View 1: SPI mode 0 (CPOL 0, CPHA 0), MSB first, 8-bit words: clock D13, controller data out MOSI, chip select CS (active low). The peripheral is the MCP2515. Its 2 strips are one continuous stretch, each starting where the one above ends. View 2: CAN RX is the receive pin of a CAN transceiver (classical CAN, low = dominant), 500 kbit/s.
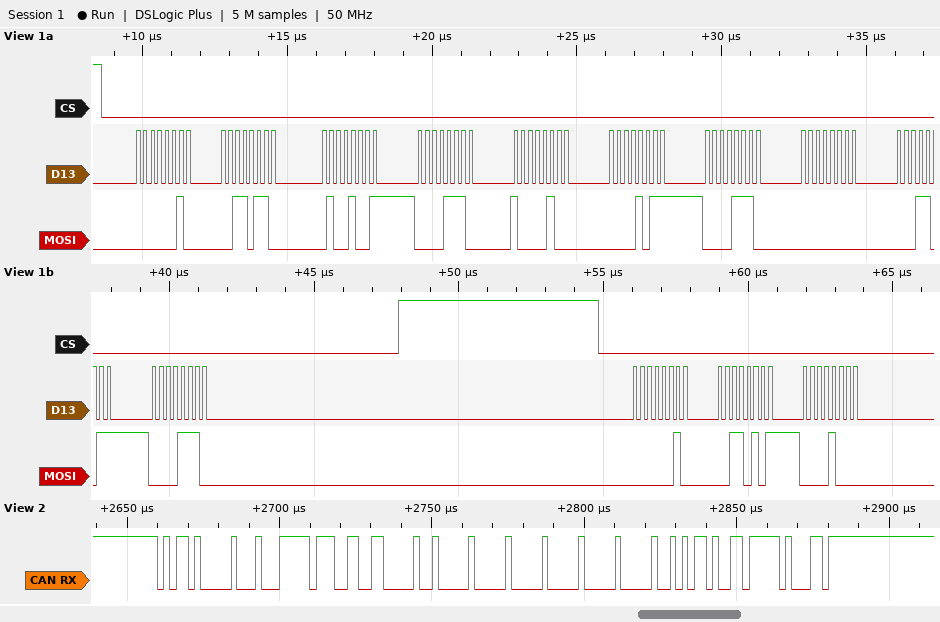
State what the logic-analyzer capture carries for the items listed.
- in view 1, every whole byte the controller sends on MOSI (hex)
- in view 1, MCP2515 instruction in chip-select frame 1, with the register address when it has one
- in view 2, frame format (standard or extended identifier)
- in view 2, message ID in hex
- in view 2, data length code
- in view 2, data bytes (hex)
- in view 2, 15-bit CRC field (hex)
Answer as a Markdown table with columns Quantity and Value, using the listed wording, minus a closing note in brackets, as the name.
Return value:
| Quantity | Value |
|---|---|
| in view 1, every whole byte the controller sends on MOSI | 02 36 49 0E 84 0B 0E 00 1B 0E 02 35 08 |
| in view 1, MCP2515 instruction in chip-select frame 1, with the register address when it has one | WRITE 0x36 |
| in view 2, frame format | standard |
| in view 2, message ID in hex | 0x5A0 |
| in view 2, data length code | 8 |
| in view 2, data bytes | FF 33 01 00 00 00 00 AD |
| in view 2, 15-bit CRC field | 0x1BF1 |
